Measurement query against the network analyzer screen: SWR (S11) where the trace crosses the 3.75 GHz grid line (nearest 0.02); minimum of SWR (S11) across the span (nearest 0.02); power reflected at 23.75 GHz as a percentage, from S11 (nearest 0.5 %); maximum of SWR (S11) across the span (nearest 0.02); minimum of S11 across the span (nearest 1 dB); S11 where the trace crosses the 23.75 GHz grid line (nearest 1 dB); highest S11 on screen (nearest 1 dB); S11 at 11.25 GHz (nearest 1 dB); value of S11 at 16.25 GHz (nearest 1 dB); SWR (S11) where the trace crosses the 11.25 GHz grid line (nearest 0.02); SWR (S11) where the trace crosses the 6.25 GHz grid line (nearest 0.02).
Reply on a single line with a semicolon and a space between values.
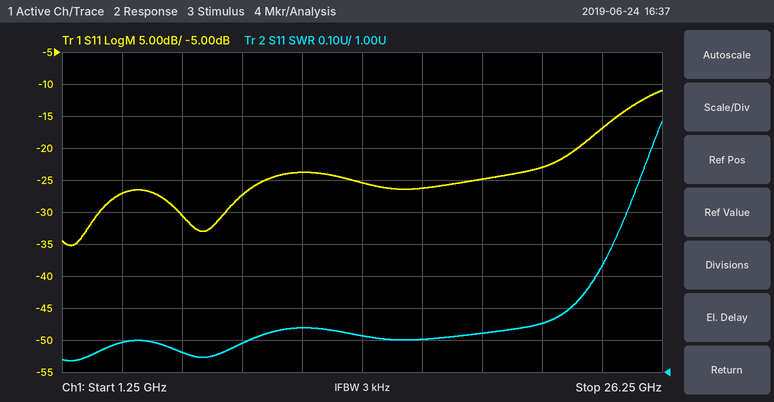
1.10; 1.04; 2.0 %; 1.78; -35 dB; -17 dB; -11 dB; -24 dB; -26 dB; 1.14; 1.06
